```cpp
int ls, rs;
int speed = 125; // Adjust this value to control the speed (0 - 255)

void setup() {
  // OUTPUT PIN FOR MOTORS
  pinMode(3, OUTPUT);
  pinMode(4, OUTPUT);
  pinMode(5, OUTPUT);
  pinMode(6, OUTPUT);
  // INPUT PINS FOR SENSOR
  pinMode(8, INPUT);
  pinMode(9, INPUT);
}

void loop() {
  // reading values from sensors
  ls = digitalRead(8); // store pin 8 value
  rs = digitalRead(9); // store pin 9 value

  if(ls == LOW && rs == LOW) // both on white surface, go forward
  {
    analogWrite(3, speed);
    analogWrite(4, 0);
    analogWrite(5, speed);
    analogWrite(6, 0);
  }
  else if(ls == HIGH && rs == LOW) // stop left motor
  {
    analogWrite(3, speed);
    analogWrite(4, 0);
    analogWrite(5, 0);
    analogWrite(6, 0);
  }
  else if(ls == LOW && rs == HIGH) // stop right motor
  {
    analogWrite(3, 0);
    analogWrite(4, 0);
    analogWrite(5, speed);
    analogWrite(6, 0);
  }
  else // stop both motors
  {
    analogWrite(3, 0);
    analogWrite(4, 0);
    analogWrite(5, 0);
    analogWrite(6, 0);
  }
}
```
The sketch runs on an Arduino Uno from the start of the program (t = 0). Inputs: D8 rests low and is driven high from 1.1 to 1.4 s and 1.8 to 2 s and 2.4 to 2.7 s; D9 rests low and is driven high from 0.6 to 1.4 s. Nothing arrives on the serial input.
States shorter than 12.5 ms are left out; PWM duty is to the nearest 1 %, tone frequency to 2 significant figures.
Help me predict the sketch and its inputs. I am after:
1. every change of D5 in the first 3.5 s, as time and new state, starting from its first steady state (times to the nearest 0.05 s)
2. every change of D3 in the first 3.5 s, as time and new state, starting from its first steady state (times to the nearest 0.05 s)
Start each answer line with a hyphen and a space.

- 0 s PWM 49 %; 1.1 s low; 1.4 s PWM 49 %; 1.8 s low; 2 s PWM 49 %; 2.4 s low; 2.7 s PWM 49 %
- 0 s PWM 49 %; 0.6 s low; 1.4 s PWM 49 %
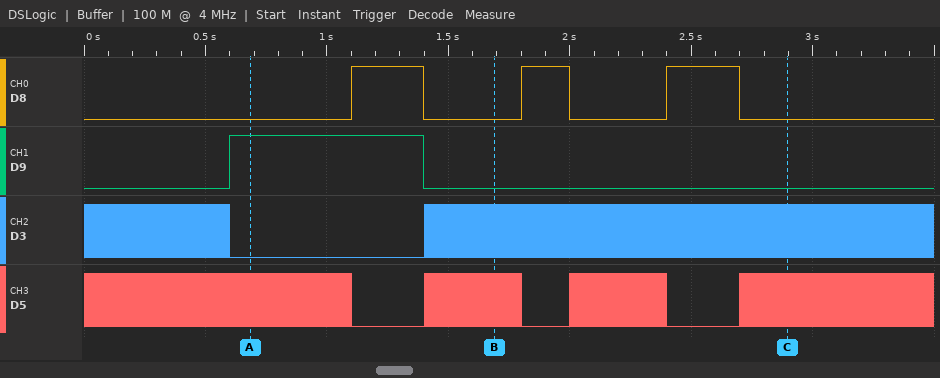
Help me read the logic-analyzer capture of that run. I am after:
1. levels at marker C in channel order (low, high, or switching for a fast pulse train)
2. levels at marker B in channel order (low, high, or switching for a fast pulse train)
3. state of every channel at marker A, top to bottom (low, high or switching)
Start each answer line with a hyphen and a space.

- D8 low, D9 low, D3 switching, D5 switching
- D8 low, D9 low, D3 switching, D5 switching
- D8 low, D9 high, D3 low, D5 switching
